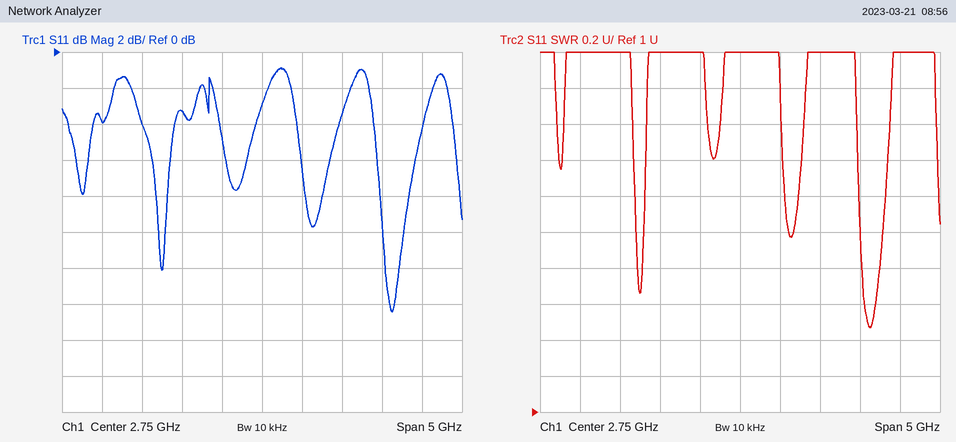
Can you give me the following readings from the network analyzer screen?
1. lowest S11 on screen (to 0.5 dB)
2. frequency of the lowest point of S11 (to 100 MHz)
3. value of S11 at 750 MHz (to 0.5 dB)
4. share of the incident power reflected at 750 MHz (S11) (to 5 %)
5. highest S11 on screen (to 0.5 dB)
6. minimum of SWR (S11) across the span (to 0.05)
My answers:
-14.5 dB
4.4 GHz
-4.0 dB
40 %
-1.0 dB
1.45
